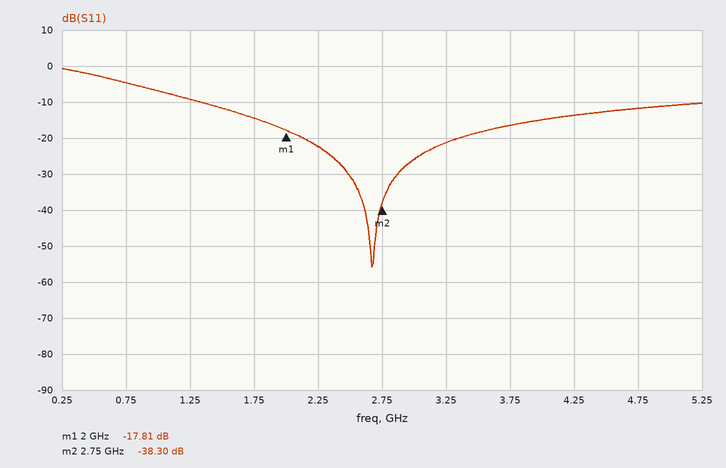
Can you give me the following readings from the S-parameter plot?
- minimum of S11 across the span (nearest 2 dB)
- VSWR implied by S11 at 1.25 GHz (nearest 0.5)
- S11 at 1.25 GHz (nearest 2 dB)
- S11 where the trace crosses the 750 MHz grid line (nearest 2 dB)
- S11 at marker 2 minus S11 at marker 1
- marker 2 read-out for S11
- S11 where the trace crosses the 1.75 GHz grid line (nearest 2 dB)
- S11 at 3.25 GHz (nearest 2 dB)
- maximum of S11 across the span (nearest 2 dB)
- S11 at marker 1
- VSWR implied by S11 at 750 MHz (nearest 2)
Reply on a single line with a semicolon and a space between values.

-56 dB; 2.0; -10 dB; -4 dB; -20.49 dB; -38.30 dB; -14 dB; -22 dB; 0 dB; -17.81 dB; 4
